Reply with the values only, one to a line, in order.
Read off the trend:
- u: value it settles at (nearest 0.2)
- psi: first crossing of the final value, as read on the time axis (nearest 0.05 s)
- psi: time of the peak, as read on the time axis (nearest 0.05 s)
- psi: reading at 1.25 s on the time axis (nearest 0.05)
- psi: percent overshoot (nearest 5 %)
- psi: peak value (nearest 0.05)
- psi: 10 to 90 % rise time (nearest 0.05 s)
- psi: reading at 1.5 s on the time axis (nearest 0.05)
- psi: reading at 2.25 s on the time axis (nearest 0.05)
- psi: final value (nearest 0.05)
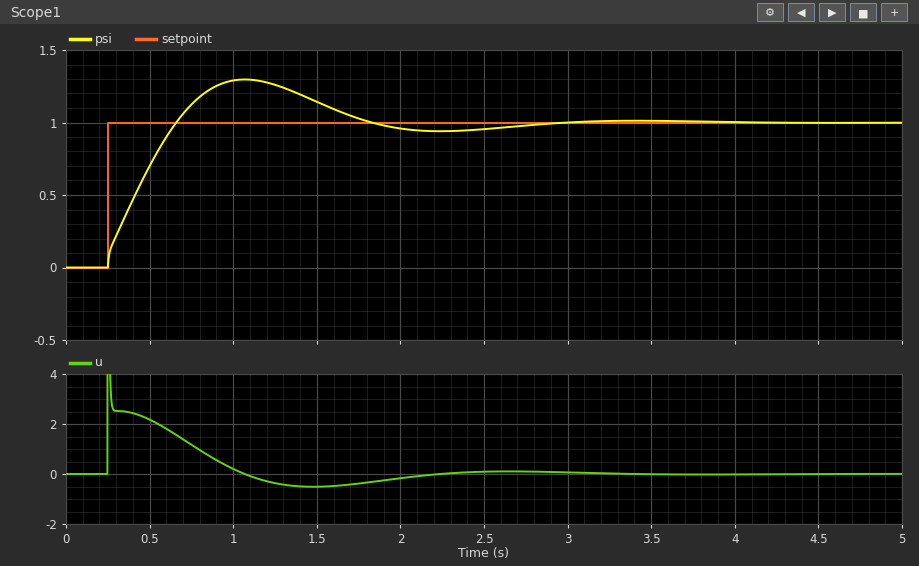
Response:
0.0
0.65 s
1.05 s
1.25
30 %
1.30
0.35 s
1.15
0.95
1.00
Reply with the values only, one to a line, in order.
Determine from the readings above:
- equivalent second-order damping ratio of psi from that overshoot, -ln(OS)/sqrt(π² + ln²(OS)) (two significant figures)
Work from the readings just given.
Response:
0.36
